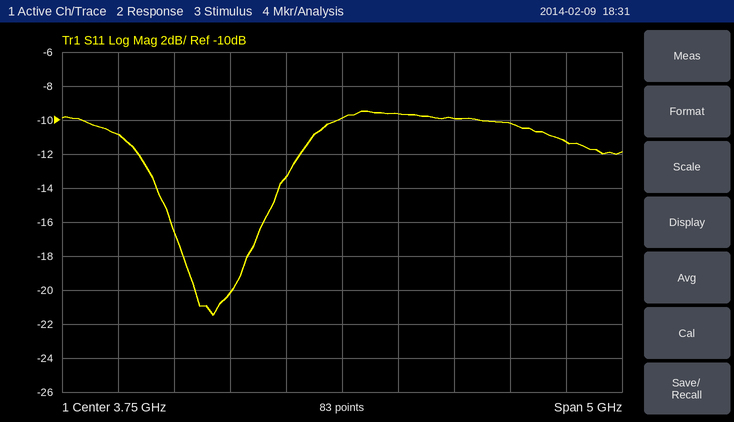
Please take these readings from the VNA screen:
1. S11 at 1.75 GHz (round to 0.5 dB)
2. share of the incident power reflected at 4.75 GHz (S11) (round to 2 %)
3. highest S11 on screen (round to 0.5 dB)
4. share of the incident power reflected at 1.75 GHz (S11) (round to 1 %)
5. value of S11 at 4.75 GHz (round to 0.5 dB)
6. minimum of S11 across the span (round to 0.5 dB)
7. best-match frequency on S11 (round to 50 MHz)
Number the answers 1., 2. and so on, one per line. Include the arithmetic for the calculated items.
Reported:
1. -11.0 dB
2. 10^(-10/10) ≈ 10 %
3. -9.5 dB
4. 10^(-11/10) ≈ 8 %
5. -10.0 dB
6. -21.5 dB
7. 2.60 GHz
